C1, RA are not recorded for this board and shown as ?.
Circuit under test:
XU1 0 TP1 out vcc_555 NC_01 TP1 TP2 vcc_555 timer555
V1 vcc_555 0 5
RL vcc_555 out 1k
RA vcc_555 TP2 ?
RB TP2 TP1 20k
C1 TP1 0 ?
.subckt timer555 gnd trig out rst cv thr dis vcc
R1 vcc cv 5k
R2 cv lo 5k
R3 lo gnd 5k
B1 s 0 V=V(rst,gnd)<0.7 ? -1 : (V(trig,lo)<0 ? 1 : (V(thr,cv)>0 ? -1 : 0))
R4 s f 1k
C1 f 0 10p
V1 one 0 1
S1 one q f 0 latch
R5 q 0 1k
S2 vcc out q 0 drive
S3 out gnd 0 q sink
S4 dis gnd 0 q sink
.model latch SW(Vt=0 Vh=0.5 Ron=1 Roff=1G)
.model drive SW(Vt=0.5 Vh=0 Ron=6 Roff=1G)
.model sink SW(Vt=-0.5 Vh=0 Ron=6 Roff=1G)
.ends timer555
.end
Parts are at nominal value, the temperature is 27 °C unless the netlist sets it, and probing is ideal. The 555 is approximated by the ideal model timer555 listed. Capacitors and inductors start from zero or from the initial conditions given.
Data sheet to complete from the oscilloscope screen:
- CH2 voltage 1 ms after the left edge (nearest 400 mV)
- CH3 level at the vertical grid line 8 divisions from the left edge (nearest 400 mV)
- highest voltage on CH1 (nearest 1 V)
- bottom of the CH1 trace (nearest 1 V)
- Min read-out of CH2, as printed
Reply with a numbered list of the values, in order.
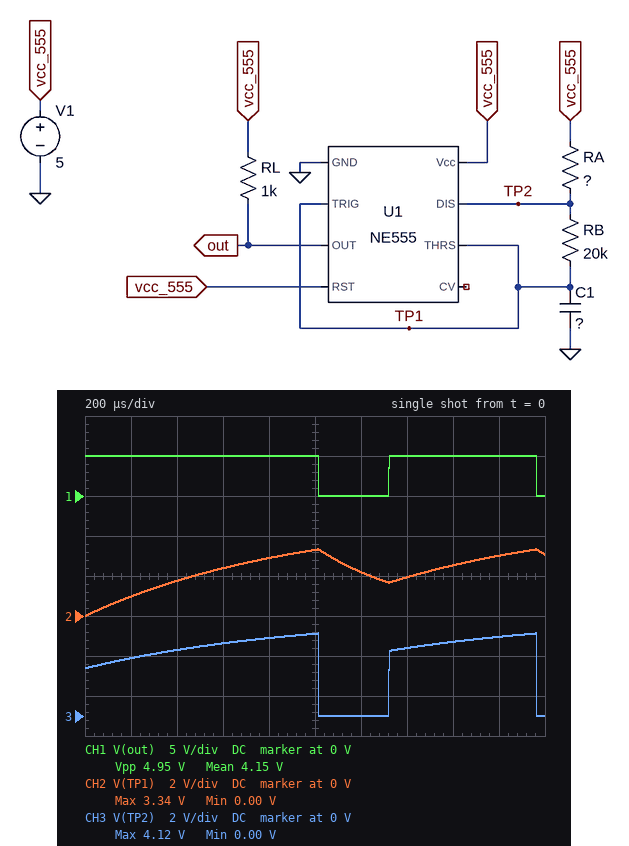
1. 3.2 V
2. 3.6 V
3. 5 V
4. 0 V
5. 0.00 V
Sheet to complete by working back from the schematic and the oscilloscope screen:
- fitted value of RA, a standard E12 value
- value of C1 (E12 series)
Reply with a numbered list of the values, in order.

1. 22 kΩ
2. 22 nF
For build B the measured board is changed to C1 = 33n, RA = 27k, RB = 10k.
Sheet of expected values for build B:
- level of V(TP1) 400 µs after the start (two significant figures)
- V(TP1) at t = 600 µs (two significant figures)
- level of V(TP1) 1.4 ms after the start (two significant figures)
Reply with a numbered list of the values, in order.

1. 1.4 V
2. 1.9 V
3. 2.8 V
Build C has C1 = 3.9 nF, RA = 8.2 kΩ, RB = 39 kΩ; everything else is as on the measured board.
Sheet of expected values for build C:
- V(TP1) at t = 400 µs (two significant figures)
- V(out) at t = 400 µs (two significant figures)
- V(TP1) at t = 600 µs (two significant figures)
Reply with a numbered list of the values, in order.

1. 3.0 V
2. 5.0 V
3. 2.6 V
